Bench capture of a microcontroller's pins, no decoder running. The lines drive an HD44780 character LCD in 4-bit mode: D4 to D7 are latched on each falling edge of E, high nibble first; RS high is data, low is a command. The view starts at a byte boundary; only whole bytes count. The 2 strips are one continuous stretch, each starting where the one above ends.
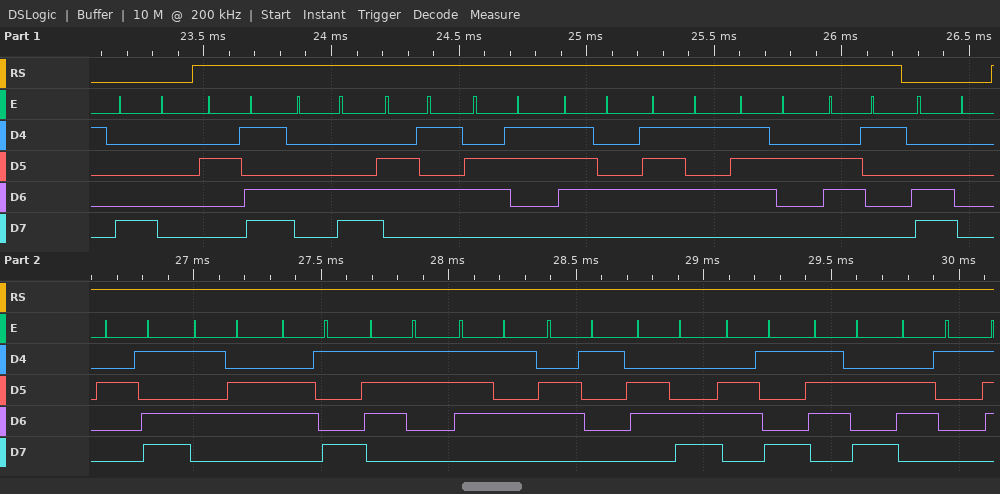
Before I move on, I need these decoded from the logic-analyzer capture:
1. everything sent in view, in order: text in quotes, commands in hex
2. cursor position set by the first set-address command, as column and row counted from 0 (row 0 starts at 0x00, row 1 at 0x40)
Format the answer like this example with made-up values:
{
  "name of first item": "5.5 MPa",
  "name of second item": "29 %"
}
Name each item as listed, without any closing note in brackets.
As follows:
{
  "everything sent in view, in order: text in quotes, commands in hex": "0x80 \"-Lectura\" 0xC0 \"-Visualiza\"",
  "cursor position set by the first set-address command, as column and row counted from 0": "column 0, row 0"
}
